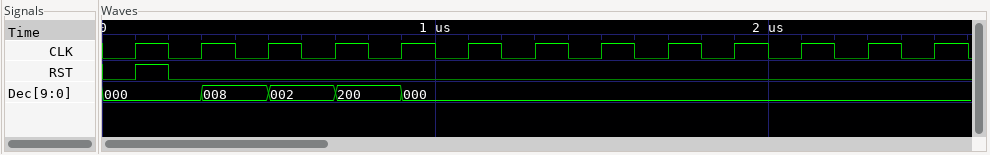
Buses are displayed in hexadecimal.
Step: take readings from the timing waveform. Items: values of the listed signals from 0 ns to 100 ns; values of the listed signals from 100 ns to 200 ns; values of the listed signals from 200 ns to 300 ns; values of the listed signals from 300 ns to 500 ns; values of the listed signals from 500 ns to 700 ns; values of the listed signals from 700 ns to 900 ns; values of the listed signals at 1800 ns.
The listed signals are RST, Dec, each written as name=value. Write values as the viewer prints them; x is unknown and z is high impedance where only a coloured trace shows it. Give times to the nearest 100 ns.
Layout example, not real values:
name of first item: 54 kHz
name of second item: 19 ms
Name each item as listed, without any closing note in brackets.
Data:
values of the listed signals from 0 ns to 100 ns: RST=0, Dec=000
values of the listed signals from 100 ns to 200 ns: RST=1, Dec=000
values of the listed signals from 200 ns to 300 ns: RST=0, Dec=000
values of the listed signals from 300 ns to 500 ns: RST=0, Dec=008
values of the listed signals from 500 ns to 700 ns: RST=0, Dec=002
values of the listed signals from 700 ns to 900 ns: RST=0, Dec=200
values of the listed signals at 1800 ns: RST=0, Dec=000
